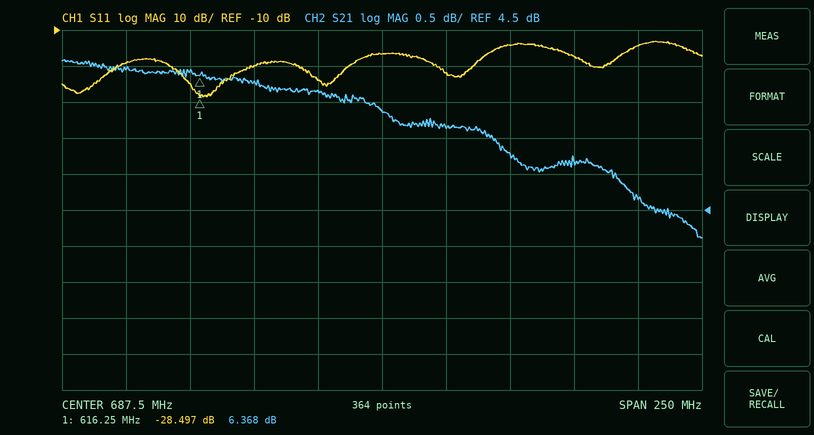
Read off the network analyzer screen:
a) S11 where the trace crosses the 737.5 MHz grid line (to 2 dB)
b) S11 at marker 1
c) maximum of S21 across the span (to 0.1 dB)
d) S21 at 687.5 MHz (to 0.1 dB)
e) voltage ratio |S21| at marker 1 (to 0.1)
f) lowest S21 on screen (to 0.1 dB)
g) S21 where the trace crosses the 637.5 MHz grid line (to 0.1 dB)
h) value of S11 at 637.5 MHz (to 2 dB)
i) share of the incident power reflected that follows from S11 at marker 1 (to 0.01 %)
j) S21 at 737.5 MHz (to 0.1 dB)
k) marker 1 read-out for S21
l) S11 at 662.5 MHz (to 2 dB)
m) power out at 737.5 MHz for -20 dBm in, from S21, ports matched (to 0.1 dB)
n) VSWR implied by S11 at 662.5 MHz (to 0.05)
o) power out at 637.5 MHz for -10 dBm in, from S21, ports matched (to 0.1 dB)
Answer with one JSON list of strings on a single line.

["-14 dB", "-28.497 dB", "6.6 dB", "5.9 dB", "2.1", "4.1 dB", "6.3 dB", "-20 dB", "0.14 %", "5.3 dB", "6.368 dB", "-24 dB", "-14.7 dBm", "1.15", "-3.7 dBm"]
